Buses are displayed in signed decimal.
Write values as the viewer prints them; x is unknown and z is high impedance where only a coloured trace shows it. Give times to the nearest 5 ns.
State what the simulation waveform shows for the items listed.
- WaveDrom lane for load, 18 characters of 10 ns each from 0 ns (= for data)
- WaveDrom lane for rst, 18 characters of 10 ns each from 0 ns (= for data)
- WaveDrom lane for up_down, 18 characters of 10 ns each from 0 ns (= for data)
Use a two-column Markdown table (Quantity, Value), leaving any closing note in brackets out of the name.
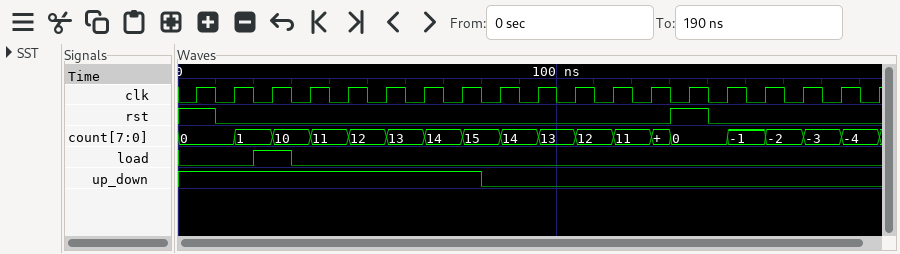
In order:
| Quantity | Value |
|---|---|
| WaveDrom lane for load, 18 characters of 10 ns each from 0 ns | {name: 'load', wave: '0.10..............'} |
| WaveDrom lane for rst, 18 characters of 10 ns each from 0 ns | {name: 'rst', wave: '10...........10...'} |
| WaveDrom lane for up_down, 18 characters of 10 ns each from 0 ns | {name: 'up_down', wave: '1.......0.........'} |
